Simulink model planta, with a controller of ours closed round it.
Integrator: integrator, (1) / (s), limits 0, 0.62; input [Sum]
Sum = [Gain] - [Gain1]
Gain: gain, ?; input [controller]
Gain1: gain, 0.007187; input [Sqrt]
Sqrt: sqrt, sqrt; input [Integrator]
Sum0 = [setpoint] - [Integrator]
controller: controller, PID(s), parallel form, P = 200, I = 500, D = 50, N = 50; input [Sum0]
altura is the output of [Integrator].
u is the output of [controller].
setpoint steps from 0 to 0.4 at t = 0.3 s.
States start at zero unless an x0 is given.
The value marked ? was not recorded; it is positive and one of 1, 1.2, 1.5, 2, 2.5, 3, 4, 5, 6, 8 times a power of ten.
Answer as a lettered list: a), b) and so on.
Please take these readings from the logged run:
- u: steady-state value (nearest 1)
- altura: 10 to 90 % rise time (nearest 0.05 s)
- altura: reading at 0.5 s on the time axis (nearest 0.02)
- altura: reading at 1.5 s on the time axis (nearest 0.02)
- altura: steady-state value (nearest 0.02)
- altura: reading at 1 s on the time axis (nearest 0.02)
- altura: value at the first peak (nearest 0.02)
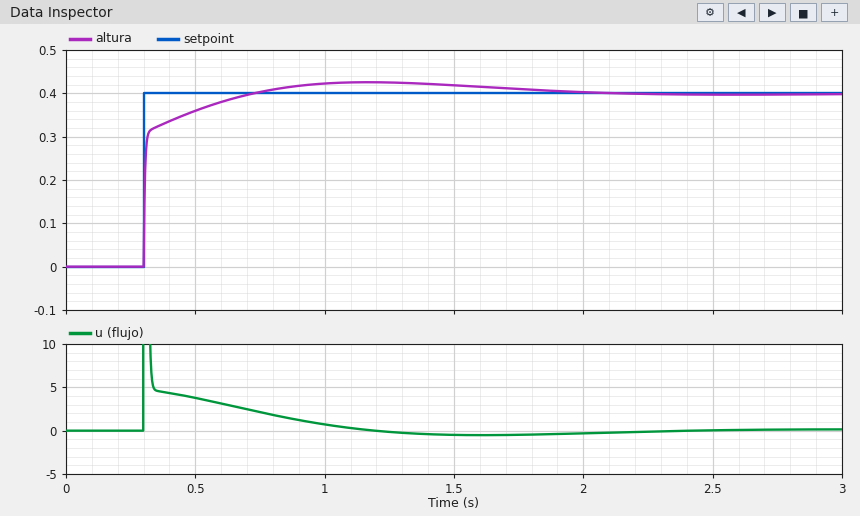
a) 0
b) 0.20 s
c) 0.36
d) 0.42
e) 0.40
f) 0.42
g) 0.42
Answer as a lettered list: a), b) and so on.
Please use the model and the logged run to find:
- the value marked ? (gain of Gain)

a) 0.06
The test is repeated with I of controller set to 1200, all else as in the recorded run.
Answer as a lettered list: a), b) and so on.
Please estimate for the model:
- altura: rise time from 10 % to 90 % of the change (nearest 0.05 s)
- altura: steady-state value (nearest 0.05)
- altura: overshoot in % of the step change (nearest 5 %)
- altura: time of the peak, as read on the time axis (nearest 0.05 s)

a) 0.15 s
b) 0.40
c) 10 %
d) 0.90 s
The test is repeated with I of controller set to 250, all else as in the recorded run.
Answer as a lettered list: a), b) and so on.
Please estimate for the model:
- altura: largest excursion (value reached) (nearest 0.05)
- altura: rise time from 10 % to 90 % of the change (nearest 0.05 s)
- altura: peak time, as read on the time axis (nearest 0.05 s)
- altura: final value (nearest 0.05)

a) 0.40
b) 0.25 s
c) 1.45 s
d) 0.40
